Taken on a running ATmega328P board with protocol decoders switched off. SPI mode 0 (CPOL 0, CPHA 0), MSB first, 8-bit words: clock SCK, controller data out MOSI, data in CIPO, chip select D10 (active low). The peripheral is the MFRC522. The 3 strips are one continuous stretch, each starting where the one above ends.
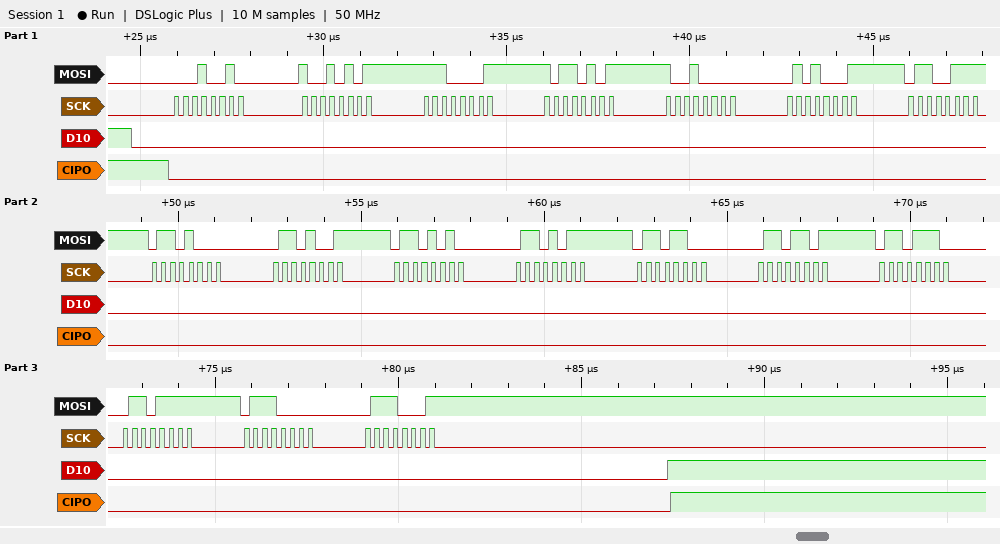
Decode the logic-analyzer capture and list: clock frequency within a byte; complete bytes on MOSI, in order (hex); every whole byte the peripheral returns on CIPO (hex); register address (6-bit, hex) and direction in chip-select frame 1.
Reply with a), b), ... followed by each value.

a) 4 MHz
b) 12 95 E1 B5 90 51 67 68 69 6A 6B 6C 6D 6E 6F 70 71
c) 00 00 00 00 00 00 00 00 00 00 00 00 00 00 00 00 00
d) 0x09 write
